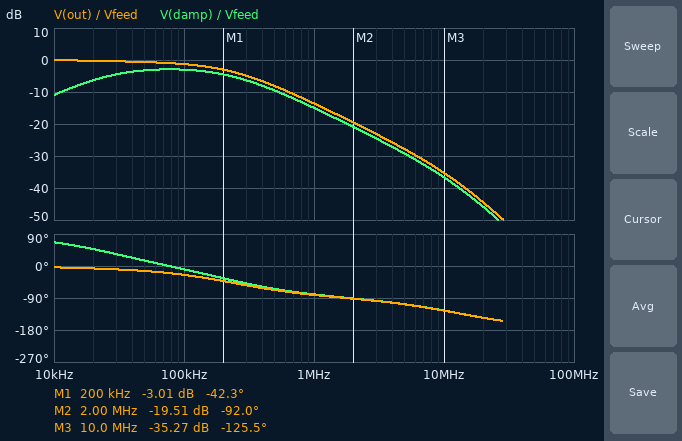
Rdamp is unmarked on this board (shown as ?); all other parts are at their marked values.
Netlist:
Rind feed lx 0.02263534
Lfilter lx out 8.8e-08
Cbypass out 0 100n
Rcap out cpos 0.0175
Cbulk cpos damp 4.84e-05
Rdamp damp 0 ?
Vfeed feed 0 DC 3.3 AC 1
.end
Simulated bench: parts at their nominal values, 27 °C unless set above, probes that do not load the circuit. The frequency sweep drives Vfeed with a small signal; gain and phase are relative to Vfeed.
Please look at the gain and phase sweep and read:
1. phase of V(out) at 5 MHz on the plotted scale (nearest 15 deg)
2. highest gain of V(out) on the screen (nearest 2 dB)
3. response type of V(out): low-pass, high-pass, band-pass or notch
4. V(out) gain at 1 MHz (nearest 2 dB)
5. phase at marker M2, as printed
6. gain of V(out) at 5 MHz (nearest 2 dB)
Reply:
-105 deg
0 dB
low-pass
-14 dB
-92.0 deg
-28 dB
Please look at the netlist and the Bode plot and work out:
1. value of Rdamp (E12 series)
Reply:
0.1 Ω
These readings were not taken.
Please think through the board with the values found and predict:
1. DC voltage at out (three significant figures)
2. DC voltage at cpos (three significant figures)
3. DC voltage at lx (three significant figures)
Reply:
3.30 V
3.30 V
3.30 V
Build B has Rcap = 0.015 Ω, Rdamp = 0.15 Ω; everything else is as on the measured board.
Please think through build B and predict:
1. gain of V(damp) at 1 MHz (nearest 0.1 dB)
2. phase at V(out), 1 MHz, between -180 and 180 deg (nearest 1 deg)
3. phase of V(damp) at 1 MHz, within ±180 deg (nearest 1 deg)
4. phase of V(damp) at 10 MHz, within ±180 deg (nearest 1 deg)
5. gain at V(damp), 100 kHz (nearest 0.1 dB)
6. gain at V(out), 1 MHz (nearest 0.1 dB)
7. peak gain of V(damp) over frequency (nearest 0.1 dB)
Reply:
-11.6 dB
-78 deg
-77 deg
-135 deg
-2.0 dB
-10.7 dB
-1.9 dB
